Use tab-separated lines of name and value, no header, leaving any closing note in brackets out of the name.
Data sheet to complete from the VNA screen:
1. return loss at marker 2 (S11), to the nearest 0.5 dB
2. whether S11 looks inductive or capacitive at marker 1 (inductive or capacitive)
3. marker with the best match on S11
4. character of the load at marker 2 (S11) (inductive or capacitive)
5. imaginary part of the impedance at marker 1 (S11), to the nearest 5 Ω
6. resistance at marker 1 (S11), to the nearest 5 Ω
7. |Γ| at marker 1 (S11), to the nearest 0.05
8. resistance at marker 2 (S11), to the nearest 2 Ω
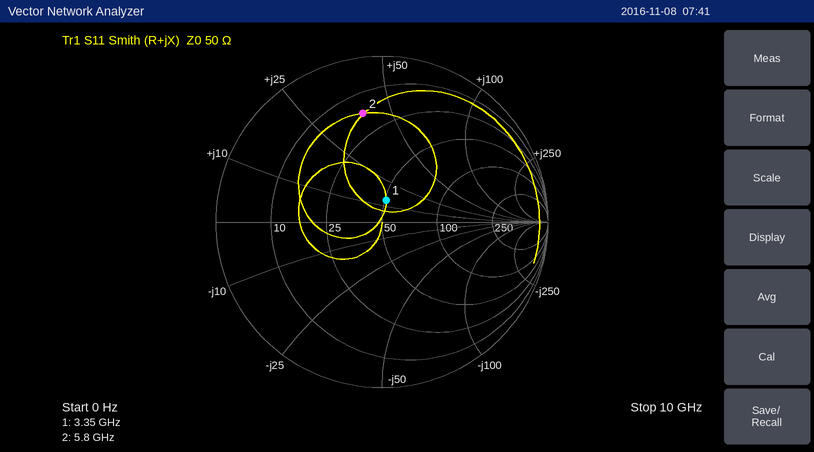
return loss at marker 2 (S11), to the nearest 0.5 dB	3.5 dB
whether S11 looks inductive or capacitive at marker 1	inductive
marker with the best match on S11	marker 1
character of the load at marker 2 (S11)	inductive
imaginary part of the impedance at marker 1 (S11), to the nearest 5 Ω	+15 Ω
resistance at marker 1 (S11), to the nearest 5 Ω	50 Ω
|Γ| at marker 1 (S11), to the nearest 0.05	0.15
resistance at marker 2 (S11), to the nearest 2 Ω	16 Ω
